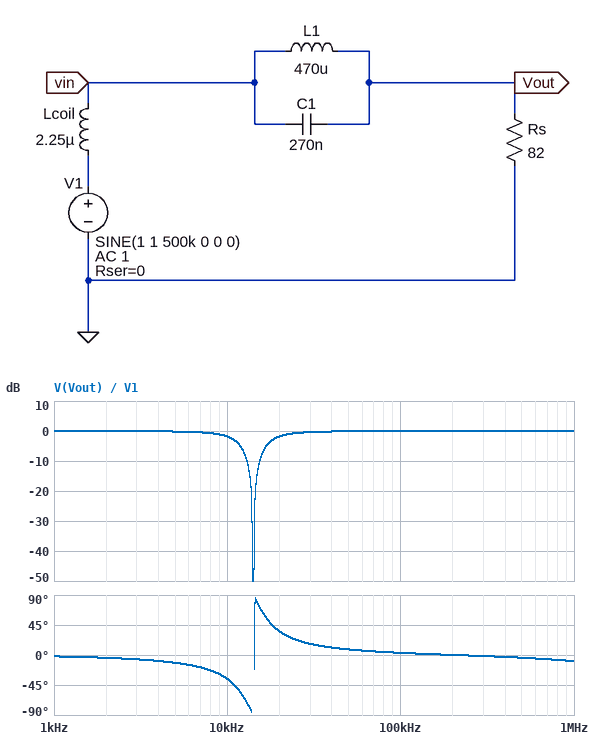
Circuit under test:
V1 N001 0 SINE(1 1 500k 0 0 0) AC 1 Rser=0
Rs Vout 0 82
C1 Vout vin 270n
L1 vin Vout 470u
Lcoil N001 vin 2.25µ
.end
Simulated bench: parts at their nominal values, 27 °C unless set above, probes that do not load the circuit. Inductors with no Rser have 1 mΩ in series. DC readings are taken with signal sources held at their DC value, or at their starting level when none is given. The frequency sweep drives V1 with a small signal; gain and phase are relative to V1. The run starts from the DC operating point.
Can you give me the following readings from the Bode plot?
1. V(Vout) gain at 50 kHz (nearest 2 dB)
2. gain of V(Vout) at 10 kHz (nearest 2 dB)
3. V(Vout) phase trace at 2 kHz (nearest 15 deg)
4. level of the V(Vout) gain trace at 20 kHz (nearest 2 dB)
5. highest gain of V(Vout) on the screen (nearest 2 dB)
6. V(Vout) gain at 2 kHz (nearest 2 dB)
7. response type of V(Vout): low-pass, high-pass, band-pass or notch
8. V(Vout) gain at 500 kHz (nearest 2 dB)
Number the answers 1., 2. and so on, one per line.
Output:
1. 0 dB
2. -2 dB
3. 0 deg
4. -2 dB
5. 0 dB
6. 0 dB
7. notch
8. 0 dB
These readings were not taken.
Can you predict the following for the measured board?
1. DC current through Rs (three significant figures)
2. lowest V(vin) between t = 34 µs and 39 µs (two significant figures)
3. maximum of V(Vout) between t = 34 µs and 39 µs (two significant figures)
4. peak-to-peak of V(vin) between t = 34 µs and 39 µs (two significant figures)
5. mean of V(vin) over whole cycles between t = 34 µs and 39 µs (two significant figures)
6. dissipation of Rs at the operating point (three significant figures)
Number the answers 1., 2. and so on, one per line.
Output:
1. 12.2 mA
2. 2.5 mV
3. 2.0 V
4. 2.0 V
5. 1.0 V
6. 12.2 mW
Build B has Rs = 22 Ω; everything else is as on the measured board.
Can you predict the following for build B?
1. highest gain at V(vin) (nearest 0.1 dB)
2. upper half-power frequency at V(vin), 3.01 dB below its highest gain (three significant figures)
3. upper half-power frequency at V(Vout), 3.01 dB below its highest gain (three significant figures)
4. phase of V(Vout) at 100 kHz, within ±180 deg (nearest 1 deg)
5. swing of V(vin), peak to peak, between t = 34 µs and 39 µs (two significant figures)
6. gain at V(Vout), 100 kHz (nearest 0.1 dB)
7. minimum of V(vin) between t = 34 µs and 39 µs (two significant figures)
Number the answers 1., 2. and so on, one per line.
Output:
1. 0.1 dB
2. 1.54 MHz
3. 1.58 MHz
4. 12 deg
5. 1.9 V
6. -0.2 dB
7. 33 mV
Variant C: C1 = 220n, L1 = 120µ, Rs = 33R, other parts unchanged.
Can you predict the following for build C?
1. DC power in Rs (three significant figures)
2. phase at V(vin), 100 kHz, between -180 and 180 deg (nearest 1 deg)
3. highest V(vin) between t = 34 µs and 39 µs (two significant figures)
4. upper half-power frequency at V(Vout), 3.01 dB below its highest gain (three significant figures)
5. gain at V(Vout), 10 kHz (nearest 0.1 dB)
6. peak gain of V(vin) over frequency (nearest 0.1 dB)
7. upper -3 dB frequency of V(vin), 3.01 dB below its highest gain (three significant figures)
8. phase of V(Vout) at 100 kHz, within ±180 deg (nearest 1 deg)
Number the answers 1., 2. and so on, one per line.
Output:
1. 30.3 mW
2. -2 deg
3. 2.0 V
4. 2.36 MHz
5. -0.3 dB
6. 0.1 dB
7. 2.31 MHz
8. 11 deg
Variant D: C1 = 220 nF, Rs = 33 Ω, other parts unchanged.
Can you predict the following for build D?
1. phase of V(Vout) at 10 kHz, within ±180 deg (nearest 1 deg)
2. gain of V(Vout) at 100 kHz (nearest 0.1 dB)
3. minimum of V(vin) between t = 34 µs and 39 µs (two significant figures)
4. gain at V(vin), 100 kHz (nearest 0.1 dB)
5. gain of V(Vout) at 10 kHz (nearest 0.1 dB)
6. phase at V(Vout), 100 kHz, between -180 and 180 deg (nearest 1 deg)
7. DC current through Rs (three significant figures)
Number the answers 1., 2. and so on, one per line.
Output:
1. -57 deg
2. -0.1 dB
3. 13 mV
4. 0.1 dB
5. -5.2 dB
6. 10 deg
7. 30.3 mA
